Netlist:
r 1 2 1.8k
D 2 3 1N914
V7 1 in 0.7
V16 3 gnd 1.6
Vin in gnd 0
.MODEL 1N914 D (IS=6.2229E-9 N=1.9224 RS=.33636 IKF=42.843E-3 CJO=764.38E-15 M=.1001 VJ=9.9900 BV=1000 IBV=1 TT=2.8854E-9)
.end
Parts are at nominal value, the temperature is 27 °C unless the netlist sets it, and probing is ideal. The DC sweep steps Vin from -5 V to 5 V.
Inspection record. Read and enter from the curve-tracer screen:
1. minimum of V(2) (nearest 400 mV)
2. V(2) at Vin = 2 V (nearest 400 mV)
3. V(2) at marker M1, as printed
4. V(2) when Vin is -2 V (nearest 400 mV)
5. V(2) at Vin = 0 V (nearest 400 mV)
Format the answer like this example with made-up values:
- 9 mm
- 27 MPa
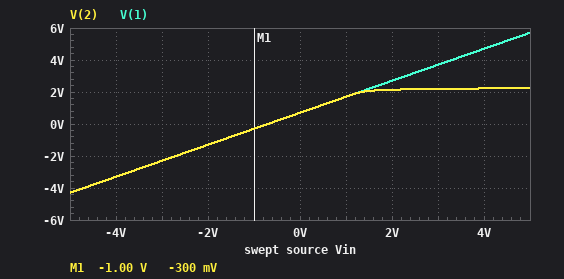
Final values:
- -4.4 V
- 2.0 V
- -300 mV
- -1.2 V
- 800 mV
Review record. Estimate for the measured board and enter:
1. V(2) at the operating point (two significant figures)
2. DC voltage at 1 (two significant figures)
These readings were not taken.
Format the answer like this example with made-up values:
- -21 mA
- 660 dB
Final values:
- 700 mV
- 700 mV
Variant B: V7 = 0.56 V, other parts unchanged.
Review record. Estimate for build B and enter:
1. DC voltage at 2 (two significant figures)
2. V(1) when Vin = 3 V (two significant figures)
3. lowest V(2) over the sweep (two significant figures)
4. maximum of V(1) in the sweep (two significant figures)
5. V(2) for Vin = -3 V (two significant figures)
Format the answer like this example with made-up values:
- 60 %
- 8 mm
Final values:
- 560 mV
- 3.6 V
- -4.4 V
- 5.6 V
- -2.4 V
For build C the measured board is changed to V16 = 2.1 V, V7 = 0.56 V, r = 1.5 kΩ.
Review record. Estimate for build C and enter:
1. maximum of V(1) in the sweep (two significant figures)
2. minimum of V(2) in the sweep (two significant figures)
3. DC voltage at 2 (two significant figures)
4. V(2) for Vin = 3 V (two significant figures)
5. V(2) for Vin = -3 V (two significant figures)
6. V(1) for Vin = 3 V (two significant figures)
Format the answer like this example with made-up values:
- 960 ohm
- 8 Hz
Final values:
- 5.6 V
- -4.4 V
- 560 mV
- 2.7 V
- -2.4 V
- 3.6 V
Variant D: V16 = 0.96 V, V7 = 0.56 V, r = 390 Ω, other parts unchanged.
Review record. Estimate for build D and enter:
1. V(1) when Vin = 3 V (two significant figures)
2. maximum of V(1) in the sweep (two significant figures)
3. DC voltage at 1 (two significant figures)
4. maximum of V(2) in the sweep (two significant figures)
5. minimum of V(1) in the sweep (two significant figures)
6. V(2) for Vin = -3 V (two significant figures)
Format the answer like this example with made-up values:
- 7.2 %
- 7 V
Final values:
- 3.6 V
- 5.6 V
- 560 mV
- 1.7 V
- -4.4 V
- -2.4 V
